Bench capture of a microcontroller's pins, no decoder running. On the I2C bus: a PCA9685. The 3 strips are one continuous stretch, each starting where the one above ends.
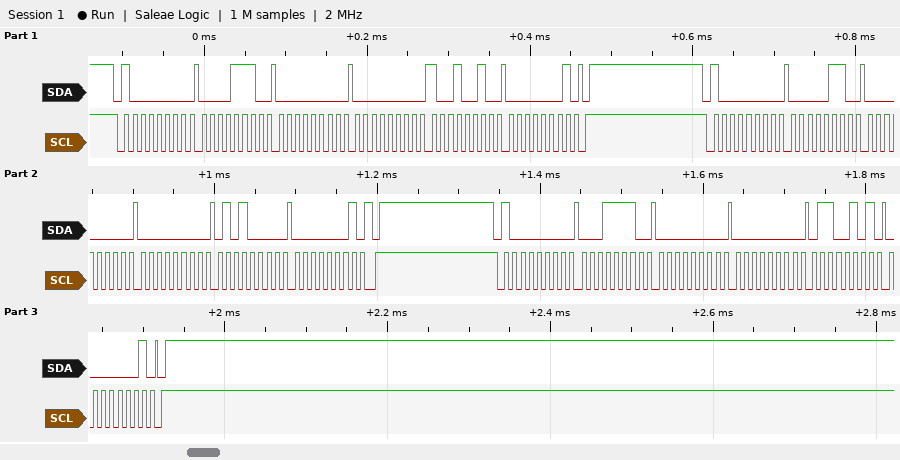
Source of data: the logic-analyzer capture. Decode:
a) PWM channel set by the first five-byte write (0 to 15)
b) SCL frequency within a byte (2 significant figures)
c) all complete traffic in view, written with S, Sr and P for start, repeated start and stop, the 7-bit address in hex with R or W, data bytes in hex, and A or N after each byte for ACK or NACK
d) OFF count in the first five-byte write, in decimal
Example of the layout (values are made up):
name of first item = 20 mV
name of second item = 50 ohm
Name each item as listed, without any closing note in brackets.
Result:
PWM channel set by the first five-byte write = 2
SCL frequency within a byte = 100 kHz
all complete traffic in view, written with S, Sr and P for start, repeated start and stop, the 7-bit address in hex with R or W, data bytes in hex, and A or N after each byte for ACK or NACK = S 40W A 0E A 00 A 00 A 92 A 01 A P S 40W A 06 A 00 A 00 A 50 A 01 A P S 40W A 1E A 00 A 00 A 65 A 01 A P
OFF count in the first five-byte write, in decimal = 402
